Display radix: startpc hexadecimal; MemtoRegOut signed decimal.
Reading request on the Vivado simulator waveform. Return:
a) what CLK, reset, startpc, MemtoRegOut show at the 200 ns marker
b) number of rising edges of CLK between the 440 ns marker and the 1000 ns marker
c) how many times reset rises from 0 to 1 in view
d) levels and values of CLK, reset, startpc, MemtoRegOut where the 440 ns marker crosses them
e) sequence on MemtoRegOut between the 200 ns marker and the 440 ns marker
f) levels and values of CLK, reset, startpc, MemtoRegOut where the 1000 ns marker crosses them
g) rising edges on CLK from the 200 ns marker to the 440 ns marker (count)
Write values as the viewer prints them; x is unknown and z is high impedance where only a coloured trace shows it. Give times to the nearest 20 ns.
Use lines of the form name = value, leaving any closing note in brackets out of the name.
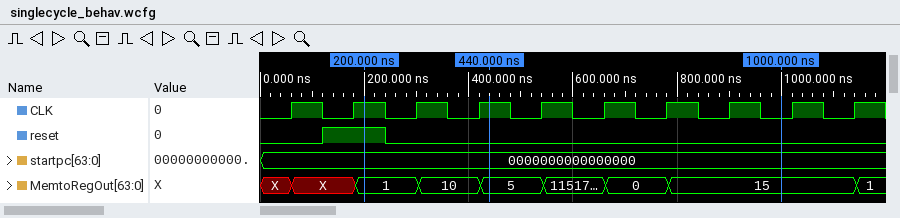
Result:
what CLK, reset, startpc, MemtoRegOut show at the 200 ns marker = CLK=1, reset=1, startpc=0000000000000000, MemtoRegOut=1
number of rising edges of CLK between the 440 ns marker and the 1000 ns marker = 4
how many times reset rises from 0 to 1 in view = 1
levels and values of CLK, reset, startpc, MemtoRegOut where the 440 ns marker crosses them = CLK=1, reset=0, startpc=0000000000000000, MemtoRegOut=5
sequence on MemtoRegOut between the 200 ns marker and the 440 ns marker = 1, 10, 5
levels and values of CLK, reset, startpc, MemtoRegOut where the 1000 ns marker crosses them = CLK=0, reset=0, startpc=0000000000000000, MemtoRegOut=15
rising edges on CLK from the 200 ns marker to the 440 ns marker = 2
